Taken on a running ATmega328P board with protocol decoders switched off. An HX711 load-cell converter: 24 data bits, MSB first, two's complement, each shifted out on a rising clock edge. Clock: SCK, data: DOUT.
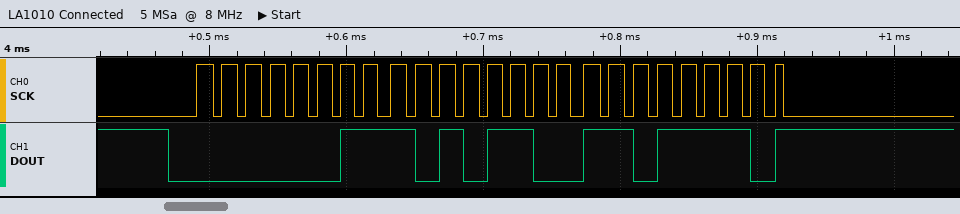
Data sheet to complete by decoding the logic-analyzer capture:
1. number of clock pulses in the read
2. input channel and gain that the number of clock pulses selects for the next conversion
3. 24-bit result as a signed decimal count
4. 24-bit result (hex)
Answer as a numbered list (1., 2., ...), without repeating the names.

1. 25
2. channel A, gain 128
3. 240862
4. 0x03ACDE
